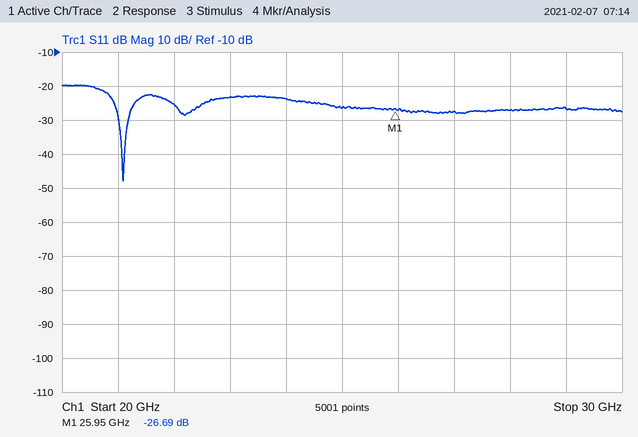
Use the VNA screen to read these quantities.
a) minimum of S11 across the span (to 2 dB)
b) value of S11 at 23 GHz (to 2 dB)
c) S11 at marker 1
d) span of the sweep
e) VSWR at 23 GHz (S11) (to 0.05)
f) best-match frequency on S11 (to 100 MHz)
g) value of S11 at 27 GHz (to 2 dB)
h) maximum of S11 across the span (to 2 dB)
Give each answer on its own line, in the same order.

-48 dB
-24 dB
-26.69 dB
10 GHz
1.15
21.1 GHz
-28 dB
-20 dB
